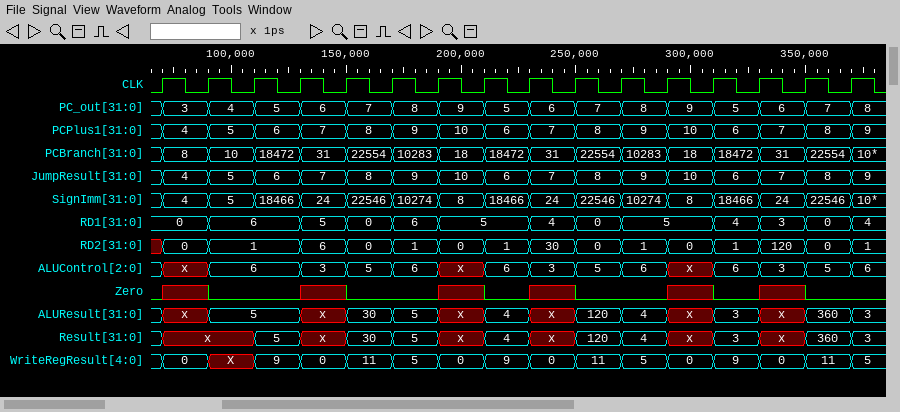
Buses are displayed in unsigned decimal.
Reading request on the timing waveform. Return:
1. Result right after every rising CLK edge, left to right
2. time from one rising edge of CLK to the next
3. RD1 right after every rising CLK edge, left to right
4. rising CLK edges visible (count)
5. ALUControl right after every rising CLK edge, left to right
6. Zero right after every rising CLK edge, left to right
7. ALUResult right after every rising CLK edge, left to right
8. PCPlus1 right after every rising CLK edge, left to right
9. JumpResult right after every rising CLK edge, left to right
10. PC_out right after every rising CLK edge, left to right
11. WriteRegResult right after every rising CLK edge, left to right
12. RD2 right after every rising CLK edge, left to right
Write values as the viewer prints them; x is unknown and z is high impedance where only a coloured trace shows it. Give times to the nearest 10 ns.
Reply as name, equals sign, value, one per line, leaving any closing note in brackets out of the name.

Result right after every rising CLK edge, left to right = x, x, 5, x, 30, 5, x, 4, x, 120, 4, x, 3, x, 360, 3
time from one rising edge of CLK to the next = 20 ns
RD1 right after every rising CLK edge, left to right = 0, 6, 6, 5, 0, 6, 5, 5, 4, 0, 5, 5, 4, 3, 0, 4
rising CLK edges visible = 16
ALUControl right after every rising CLK edge, left to right = x, 6, 6, 3, 5, 6, x, 6, 3, 5, 6, x, 6, 3, 5, 6
Zero right after every rising CLK edge, left to right = x 0 0 x 0 0 x 0 x 0 0 x 0 x 0 0
ALUResult right after every rising CLK edge, left to right = x, 5, 5, x, 30, 5, x, 4, x, 120, 4, x, 3, x, 360, 3
PCPlus1 right after every rising CLK edge, left to right = 4, 5, 6, 7, 8, 9, 10, 6, 7, 8, 9, 10, 6, 7, 8, 9
JumpResult right after every rising CLK edge, left to right = 4, 5, 6, 7, 8, 9, 10, 6, 7, 8, 9, 10, 6, 7, 8, 9
PC_out right after every rising CLK edge, left to right = 3, 4, 5, 6, 7, 8, 9, 5, 6, 7, 8, 9, 5, 6, 7, 8
WriteRegResult right after every rising CLK edge, left to right = 0, X, 9, 0, 11, 5, 0, 9, 0, 11, 5, 0, 9, 0, 11, 5
RD2 right after every rising CLK edge, left to right = 0, 1, 1, 6, 0, 1, 0, 1, 30, 0, 1, 0, 1, 120, 0, 1
